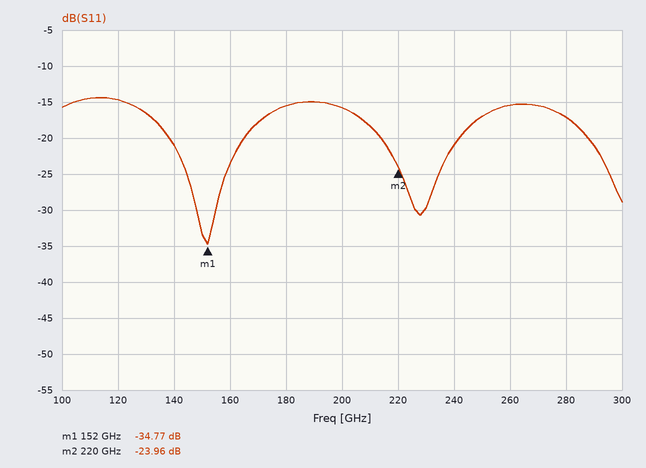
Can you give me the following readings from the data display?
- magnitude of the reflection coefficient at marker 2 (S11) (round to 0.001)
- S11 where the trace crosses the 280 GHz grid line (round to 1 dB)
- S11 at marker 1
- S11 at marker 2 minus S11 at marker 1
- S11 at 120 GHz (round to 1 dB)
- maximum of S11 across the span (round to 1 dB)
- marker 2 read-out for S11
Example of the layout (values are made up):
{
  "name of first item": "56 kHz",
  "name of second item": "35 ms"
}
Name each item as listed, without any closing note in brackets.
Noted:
{
  "magnitude of the reflection coefficient at marker 2 (S11)": "0.063",
  "S11 where the trace crosses the 280 GHz grid line": "-17 dB",
  "S11 at marker 1": "-34.77 dB",
  "S11 at marker 2 minus S11 at marker 1": "10.81 dB",
  "S11 at 120 GHz": "-15 dB",
  "maximum of S11 across the span": "-14 dB",
  "marker 2 read-out for S11": "-23.96 dB"
}
